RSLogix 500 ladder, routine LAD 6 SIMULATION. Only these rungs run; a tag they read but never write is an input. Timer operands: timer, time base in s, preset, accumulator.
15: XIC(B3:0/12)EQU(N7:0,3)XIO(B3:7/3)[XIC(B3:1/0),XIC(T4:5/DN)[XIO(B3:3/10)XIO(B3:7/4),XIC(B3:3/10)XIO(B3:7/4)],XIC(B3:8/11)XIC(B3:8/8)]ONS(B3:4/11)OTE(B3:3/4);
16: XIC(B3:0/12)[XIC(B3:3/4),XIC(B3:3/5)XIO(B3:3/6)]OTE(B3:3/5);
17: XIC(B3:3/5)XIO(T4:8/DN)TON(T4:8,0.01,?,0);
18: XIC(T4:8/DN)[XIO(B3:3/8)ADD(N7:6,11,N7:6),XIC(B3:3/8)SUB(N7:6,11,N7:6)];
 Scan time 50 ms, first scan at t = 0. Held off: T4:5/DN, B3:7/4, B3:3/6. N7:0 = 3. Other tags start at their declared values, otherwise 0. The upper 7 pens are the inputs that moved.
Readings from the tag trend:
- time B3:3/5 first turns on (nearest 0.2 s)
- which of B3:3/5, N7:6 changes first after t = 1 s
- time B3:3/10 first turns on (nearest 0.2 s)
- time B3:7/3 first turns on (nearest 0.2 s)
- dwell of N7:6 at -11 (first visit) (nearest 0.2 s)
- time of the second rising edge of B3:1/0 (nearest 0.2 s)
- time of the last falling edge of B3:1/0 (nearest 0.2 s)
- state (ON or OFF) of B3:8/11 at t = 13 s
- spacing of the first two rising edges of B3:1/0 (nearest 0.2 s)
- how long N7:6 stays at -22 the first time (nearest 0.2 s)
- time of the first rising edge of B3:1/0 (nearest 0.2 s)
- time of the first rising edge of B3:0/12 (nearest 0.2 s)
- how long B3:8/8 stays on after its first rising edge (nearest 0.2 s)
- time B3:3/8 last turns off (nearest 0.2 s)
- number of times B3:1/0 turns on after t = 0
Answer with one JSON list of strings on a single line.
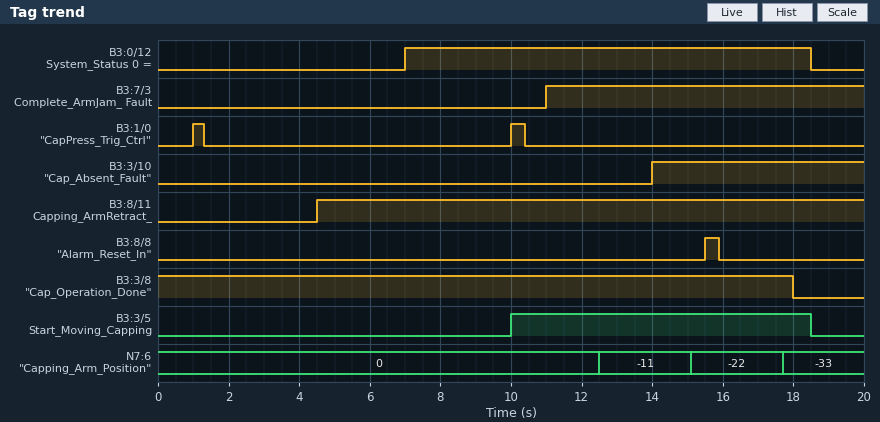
["10.0 s", "B3:3/5", "14.0 s", "11.0 s", "2.6 s", "10.0 s", "10.4 s", "ON", "9.0 s", "2.6 s", "1.0 s", "7.0 s", "0.4 s", "18.0 s", "2"]
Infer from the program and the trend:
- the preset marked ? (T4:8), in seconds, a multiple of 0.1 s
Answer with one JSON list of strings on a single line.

["2.5 s"]
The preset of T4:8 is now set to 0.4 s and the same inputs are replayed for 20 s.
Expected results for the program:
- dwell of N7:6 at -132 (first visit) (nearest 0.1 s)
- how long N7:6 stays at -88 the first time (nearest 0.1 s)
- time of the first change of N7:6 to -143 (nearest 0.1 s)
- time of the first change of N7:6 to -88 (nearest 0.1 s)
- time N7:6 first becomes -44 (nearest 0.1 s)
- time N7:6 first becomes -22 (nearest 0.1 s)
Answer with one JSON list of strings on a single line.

["0.5 s", "0.5 s", "16.4 s", "13.9 s", "11.9 s", "10.9 s"]
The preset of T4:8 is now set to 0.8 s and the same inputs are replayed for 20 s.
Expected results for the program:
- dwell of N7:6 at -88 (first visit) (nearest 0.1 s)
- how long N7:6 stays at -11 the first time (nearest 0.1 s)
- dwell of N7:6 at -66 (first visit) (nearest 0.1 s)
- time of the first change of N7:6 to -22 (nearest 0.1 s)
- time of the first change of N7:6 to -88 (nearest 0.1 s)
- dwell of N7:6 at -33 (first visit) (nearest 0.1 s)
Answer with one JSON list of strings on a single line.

["0.9 s", "0.9 s", "0.9 s", "11.7 s", "17.1 s", "0.9 s"]
